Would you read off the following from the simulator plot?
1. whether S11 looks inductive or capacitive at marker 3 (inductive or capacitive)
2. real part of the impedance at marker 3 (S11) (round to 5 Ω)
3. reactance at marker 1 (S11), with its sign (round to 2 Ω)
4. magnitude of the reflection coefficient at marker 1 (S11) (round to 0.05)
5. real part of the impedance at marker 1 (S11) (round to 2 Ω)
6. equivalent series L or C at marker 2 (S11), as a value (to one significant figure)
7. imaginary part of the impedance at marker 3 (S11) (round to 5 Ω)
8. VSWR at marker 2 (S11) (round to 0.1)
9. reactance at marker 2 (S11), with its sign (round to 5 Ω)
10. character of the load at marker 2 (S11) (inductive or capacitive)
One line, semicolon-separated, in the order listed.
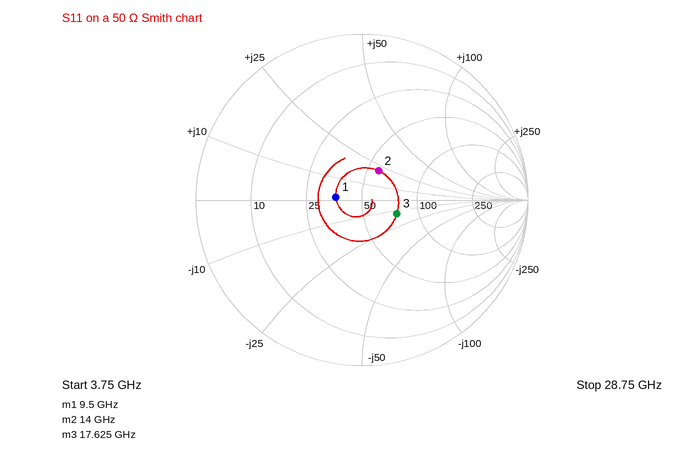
capacitive; 75 Ω; +2 Ω; 0.15; 36 Ω; 200 pH; -15 Ω; 1.5; +20 Ω; inductive
